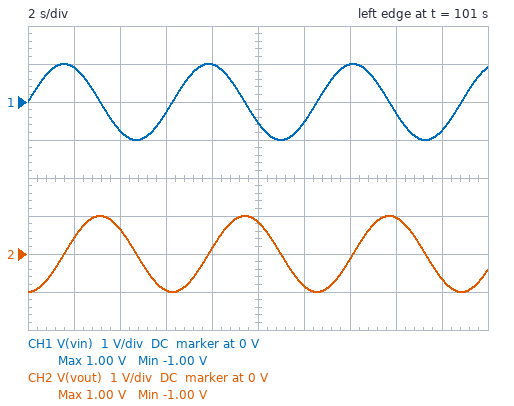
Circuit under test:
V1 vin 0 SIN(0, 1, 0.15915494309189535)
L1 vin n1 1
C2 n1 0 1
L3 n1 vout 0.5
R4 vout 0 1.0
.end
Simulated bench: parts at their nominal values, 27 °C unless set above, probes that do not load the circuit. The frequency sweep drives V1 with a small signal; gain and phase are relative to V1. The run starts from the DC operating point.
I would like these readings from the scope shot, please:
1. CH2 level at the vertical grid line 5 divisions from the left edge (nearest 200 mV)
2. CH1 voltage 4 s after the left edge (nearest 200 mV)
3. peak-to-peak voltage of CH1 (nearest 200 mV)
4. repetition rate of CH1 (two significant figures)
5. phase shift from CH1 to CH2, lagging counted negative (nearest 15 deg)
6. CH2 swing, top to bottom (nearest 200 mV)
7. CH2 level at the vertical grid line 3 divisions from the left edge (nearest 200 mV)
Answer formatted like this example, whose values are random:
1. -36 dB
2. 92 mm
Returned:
1. 800 mV
2. -800 mV
3. 2.0 V
4. 160 mHz
5. -90 deg
6. 2.0 V
7. -1.0 V
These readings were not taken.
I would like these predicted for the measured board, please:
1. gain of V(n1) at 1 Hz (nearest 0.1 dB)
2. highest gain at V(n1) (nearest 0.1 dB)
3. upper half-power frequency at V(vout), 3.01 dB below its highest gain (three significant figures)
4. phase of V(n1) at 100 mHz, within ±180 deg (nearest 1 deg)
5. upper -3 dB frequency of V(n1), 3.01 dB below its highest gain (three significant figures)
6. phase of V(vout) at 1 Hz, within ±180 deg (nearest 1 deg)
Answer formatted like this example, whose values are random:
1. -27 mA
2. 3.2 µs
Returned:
1. -31.3 dB
2. 1.1 dB
3. 242 mHz
4. -36 deg
5. 254 mHz
6. 109 deg
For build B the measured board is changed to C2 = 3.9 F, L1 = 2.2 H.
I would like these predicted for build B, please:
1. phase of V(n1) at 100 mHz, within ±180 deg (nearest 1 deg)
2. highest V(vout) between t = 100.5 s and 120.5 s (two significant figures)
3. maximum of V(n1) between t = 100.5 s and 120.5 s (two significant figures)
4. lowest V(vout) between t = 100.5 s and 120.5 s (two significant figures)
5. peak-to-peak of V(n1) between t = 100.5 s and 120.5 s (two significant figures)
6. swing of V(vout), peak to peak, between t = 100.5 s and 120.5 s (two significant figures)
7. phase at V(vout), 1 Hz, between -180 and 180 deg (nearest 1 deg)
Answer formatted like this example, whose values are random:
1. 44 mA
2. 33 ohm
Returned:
1. -148 deg
2. 130 mV
3. 140 mV
4. -130 mV
5. 290 mV
6. 260 mV
7. 108 deg
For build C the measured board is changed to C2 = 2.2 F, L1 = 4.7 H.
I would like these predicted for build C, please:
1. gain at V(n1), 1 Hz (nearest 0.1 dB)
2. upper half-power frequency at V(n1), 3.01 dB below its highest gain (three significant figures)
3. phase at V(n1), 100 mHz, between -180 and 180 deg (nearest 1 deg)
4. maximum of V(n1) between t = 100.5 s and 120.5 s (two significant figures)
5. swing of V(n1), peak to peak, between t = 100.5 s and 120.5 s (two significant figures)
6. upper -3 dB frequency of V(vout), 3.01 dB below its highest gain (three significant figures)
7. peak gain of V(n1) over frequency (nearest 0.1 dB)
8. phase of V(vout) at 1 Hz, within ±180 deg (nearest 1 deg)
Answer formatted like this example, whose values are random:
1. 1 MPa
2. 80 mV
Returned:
1. -52.0 dB
2. 48.1 mHz
3. -130 deg
4. 120 mV
5. 240 mV
6. 47.4 mHz
7. 0 dB
8. 108 deg
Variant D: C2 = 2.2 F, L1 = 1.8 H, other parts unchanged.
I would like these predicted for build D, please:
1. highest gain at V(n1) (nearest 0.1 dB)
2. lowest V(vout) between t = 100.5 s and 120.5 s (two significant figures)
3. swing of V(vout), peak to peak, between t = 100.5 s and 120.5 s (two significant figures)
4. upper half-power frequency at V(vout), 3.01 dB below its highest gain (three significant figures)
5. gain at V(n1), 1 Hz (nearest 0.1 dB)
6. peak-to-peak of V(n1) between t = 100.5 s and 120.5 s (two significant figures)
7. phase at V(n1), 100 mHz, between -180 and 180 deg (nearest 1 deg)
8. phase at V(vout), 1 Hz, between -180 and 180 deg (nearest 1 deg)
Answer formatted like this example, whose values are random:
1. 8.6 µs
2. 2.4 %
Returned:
1. 1.4 dB
2. -340 mV
3. 670 mV
4. 107 mHz
5. -43.6 dB
6. 750 mV
7. -103 deg
8. 108 deg
